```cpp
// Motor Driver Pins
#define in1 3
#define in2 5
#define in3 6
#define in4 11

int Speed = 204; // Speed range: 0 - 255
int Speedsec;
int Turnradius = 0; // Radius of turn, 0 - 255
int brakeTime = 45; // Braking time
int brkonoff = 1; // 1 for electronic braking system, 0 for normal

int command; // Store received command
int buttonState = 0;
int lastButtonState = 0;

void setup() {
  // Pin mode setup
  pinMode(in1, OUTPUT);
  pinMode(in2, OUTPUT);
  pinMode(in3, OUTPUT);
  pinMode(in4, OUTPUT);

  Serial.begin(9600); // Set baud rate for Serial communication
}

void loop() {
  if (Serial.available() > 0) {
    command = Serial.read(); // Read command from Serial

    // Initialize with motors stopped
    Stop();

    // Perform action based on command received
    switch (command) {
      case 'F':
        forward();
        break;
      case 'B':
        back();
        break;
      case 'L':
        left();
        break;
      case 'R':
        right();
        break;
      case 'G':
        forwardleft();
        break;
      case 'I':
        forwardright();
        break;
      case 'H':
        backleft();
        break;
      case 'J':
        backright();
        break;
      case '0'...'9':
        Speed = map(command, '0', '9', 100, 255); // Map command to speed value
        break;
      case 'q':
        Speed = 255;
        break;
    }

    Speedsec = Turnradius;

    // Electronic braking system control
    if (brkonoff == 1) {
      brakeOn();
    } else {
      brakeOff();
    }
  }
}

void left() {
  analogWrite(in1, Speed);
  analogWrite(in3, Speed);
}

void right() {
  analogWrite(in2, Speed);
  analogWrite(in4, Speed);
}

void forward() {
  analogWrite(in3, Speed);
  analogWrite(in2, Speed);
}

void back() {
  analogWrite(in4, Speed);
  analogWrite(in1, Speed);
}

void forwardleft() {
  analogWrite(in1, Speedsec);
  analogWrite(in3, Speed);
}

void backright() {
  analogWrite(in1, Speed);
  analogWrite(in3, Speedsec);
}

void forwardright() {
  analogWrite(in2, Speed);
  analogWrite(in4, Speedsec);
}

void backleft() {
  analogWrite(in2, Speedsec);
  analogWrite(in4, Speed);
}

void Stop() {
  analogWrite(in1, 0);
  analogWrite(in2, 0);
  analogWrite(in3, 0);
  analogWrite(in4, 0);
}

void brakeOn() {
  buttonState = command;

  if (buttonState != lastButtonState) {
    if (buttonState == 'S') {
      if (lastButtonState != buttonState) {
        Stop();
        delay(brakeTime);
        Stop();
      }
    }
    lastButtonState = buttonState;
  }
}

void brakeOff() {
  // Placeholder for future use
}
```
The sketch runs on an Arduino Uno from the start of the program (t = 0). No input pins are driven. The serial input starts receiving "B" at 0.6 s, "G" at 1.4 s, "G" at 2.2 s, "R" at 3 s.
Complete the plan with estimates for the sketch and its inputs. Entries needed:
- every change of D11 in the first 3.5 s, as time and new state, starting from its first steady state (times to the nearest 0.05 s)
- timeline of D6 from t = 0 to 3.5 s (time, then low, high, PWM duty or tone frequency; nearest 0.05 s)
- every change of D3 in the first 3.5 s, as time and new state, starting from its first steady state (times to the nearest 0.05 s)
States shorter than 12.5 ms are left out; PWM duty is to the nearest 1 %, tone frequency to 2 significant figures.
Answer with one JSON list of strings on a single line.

["0 s low; 0.6 s PWM 80 %; 1.4 s low; 3 s PWM 80 %", "0 s low; 1.4 s PWM 80 %; 3 s low", "0 s low; 0.6 s PWM 80 %; 1.4 s low"]
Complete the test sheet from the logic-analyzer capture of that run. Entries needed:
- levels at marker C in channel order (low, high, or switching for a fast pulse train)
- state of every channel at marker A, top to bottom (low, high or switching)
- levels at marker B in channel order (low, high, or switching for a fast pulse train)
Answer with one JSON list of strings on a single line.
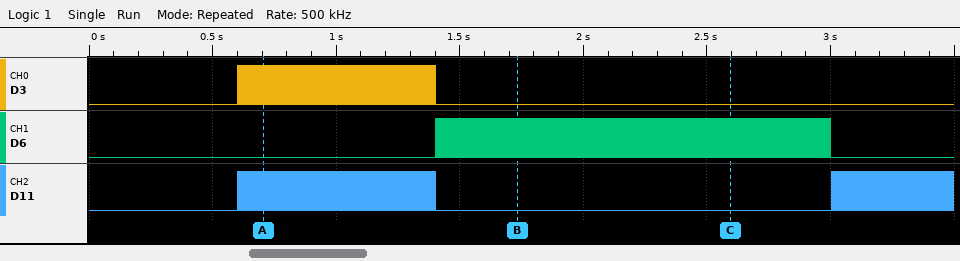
["D3 low, D6 switching, D11 low", "D3 switching, D6 low, D11 switching", "D3 low, D6 switching, D11 low"]
